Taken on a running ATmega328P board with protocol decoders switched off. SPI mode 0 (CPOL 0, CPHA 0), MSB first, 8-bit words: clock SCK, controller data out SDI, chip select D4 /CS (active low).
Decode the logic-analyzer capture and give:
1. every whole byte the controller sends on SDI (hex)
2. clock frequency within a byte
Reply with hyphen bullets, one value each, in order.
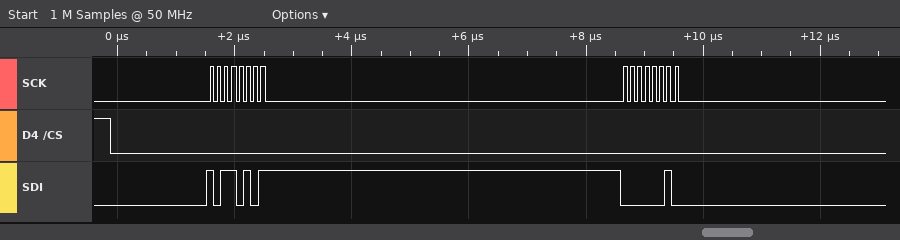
- B5 02
- 8 MHz
